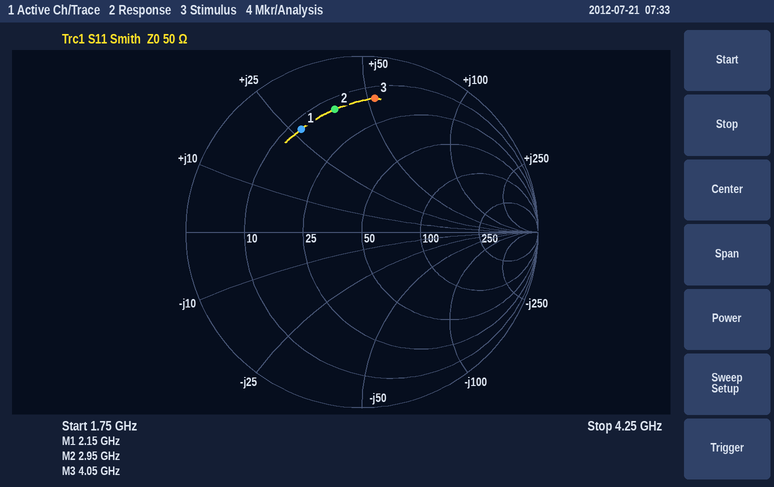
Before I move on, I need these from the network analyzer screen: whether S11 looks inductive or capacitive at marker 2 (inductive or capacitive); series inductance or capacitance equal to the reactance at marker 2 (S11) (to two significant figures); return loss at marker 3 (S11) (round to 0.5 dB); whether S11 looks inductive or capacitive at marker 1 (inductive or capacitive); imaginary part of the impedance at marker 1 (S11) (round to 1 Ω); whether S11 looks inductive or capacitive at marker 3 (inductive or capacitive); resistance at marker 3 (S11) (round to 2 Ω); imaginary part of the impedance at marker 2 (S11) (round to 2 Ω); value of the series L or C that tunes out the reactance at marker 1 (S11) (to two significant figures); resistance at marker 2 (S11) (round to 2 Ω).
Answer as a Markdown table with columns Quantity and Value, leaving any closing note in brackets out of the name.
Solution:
| Quantity | Value |
|---|---|
| whether S11 looks inductive or capacitive at marker 2 | inductive |
| series inductance or capacitance equal to the reactance at marker 2 (S11) | 2.1 nH |
| return loss at marker 3 (S11) | 2.5 dB |
| whether S11 looks inductive or capacitive at marker 1 | inductive |
| imaginary part of the impedance at marker 1 (S11) | +27 Ω |
| whether S11 looks inductive or capacitive at marker 3 | inductive |
| resistance at marker 3 (S11) | 14 Ω |
| imaginary part of the impedance at marker 2 (S11) | +38 Ω |
| value of the series L or C that tunes out the reactance at marker 1 (S11) | 2.7 pF |
| resistance at marker 2 (S11) | 14 Ω |
